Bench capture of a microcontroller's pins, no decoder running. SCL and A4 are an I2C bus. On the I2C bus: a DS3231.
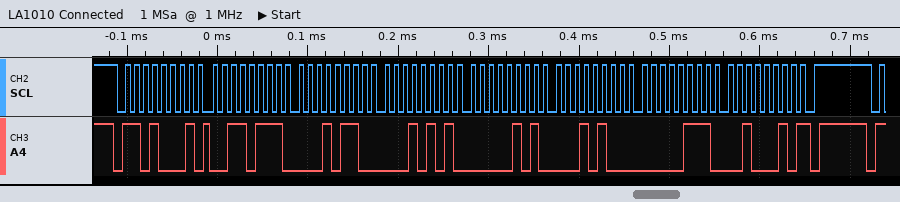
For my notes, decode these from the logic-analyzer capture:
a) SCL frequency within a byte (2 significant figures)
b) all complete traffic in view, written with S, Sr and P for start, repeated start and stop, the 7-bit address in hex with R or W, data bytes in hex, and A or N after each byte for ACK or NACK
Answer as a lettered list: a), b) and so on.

a) 100 kHz
b) S 68R A 37 A 16 A 15 A 05 A 14 A 07 A 22 N P
